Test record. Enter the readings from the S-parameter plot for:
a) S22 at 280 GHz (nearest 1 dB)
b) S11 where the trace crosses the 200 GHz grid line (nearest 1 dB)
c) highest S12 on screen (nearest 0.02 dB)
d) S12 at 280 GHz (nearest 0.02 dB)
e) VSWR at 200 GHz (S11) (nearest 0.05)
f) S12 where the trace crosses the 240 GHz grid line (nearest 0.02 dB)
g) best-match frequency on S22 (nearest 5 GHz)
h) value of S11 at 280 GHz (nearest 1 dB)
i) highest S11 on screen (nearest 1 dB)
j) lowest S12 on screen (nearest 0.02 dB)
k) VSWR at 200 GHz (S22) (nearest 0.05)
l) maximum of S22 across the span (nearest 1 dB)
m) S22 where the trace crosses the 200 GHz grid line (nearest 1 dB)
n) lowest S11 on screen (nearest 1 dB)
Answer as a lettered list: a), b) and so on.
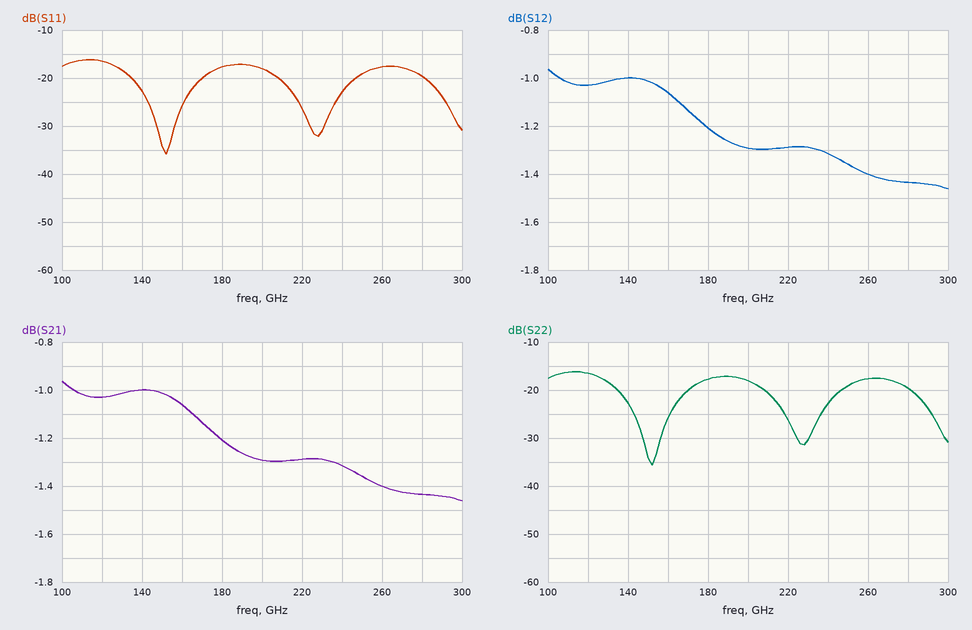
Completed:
a) -20 dB
b) -18 dB
c) -0.96 dB
d) -1.44 dB
e) 1.30
f) -1.32 dB
g) 150 GHz
h) -20 dB
i) -16 dB
j) -1.46 dB
k) 1.30
l) -16 dB
m) -18 dB
n) -36 dB
